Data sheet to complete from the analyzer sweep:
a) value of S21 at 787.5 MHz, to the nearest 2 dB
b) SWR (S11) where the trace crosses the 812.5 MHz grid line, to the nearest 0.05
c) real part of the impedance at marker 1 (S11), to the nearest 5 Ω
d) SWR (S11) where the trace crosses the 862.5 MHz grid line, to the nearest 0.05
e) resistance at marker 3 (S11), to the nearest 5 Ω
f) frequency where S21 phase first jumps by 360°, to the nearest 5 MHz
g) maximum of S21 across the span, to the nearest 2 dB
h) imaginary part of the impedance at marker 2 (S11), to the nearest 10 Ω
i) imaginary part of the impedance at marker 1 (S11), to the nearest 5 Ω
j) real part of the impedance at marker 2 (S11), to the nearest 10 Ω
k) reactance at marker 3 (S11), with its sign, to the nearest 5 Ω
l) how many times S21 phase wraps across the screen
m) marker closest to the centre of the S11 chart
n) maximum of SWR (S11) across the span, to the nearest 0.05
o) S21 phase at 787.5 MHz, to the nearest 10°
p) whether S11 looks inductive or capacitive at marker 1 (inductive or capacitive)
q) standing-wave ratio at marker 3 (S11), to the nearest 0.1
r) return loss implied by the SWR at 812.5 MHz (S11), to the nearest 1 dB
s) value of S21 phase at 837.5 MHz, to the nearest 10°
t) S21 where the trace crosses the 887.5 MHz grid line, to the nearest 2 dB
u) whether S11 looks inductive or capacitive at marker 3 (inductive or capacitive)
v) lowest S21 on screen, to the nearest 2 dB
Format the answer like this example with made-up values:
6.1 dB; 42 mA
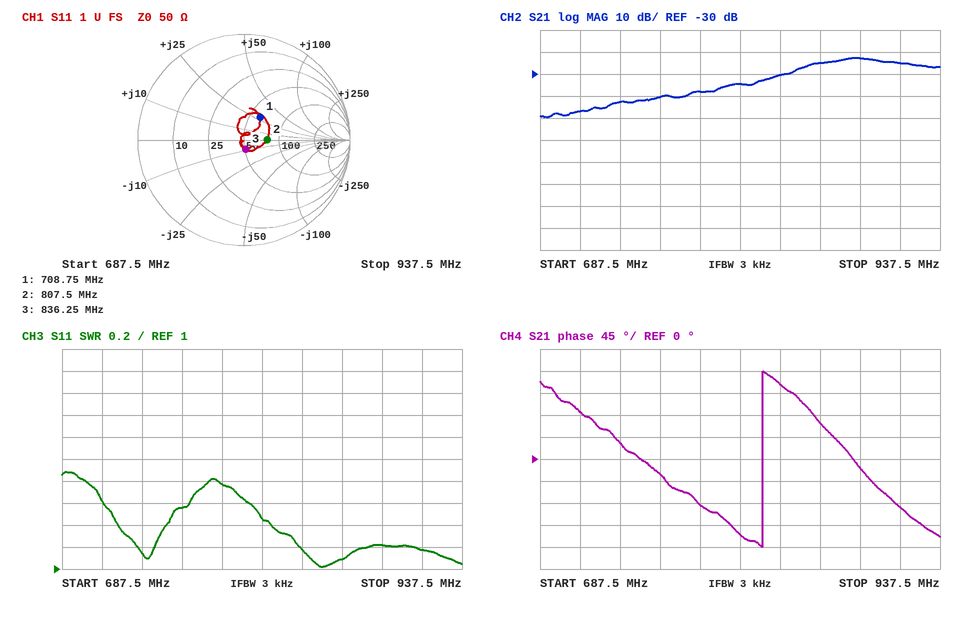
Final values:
-38 dB; 1.45; 60 Ω; 1.10; 50 Ω; 825 MHz; -22 dB; 0 Ω; +30 Ω; 80 Ω; -10 Ω; 1; marker 3; 1.90; -90°; inductive; 1.2; 15 dB; 150°; -22 dB; capacitive; -50 dB
